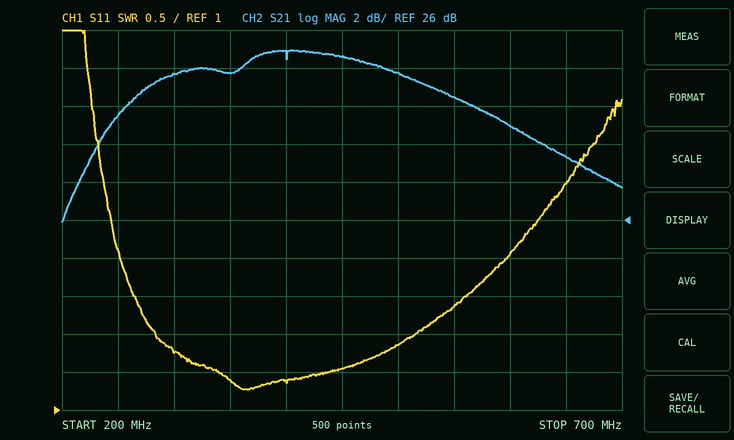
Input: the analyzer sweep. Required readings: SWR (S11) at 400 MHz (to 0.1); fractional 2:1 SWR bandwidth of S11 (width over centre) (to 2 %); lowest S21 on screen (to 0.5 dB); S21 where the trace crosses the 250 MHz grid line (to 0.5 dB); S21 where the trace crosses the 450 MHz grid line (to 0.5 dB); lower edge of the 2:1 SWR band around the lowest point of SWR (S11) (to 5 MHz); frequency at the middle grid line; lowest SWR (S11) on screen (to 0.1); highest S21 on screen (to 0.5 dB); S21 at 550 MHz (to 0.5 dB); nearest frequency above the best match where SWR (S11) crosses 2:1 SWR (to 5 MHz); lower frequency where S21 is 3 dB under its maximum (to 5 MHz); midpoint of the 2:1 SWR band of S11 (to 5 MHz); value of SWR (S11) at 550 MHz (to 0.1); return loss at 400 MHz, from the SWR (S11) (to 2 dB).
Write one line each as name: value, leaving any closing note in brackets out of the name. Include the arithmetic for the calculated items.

SWR (S11) at 400 MHz: 1.4
fractional 2:1 SWR bandwidth of S11 (width over centre): 230 MHz / 400 MHz ≈ 58 %
lowest S21 on screen: 26.0 dB
S21 where the trace crosses the 250 MHz grid line: 31.5 dB
S21 where the trace crosses the 450 MHz grid line: 34.5 dB
lower edge of the 2:1 SWR band around the lowest point of SWR (S11): 285 MHz
frequency at the middle grid line: 450 MHz
lowest SWR (S11) on screen: 1.3
highest S21 on screen: 35.0 dB
S21 at 550 MHz: 32.5 dB
nearest frequency above the best match where SWR (S11) crosses 2:1 SWR: 515 MHz
lower frequency where S21 is 3 dB under its maximum: 255 MHz
midpoint of the 2:1 SWR band of S11: 400 MHz
value of SWR (S11) at 550 MHz: 2.4
return loss at 400 MHz, from the SWR (S11): −20 log10((1.4 − 1)/(1.4 + 1)) ≈ 16 dB
